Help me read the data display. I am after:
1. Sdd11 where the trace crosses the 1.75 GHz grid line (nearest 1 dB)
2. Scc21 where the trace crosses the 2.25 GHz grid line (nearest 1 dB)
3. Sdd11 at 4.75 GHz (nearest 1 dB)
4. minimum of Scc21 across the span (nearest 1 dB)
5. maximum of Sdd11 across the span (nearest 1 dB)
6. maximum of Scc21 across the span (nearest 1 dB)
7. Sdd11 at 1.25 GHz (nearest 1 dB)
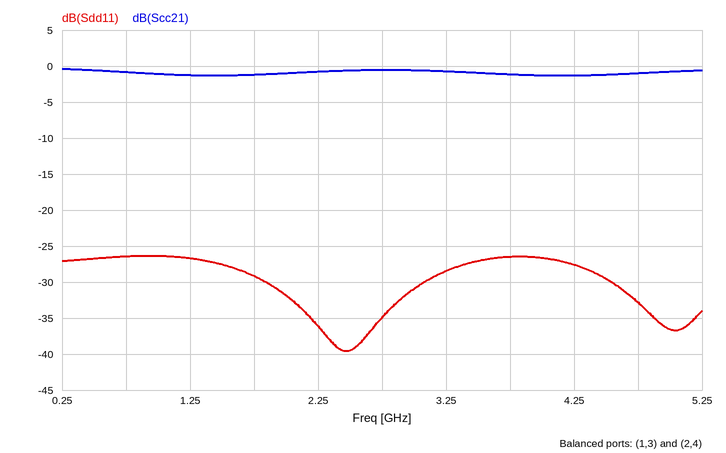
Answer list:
-29 dB
-1 dB
-33 dB
-1 dB
-26 dB
0 dB
-27 dB
